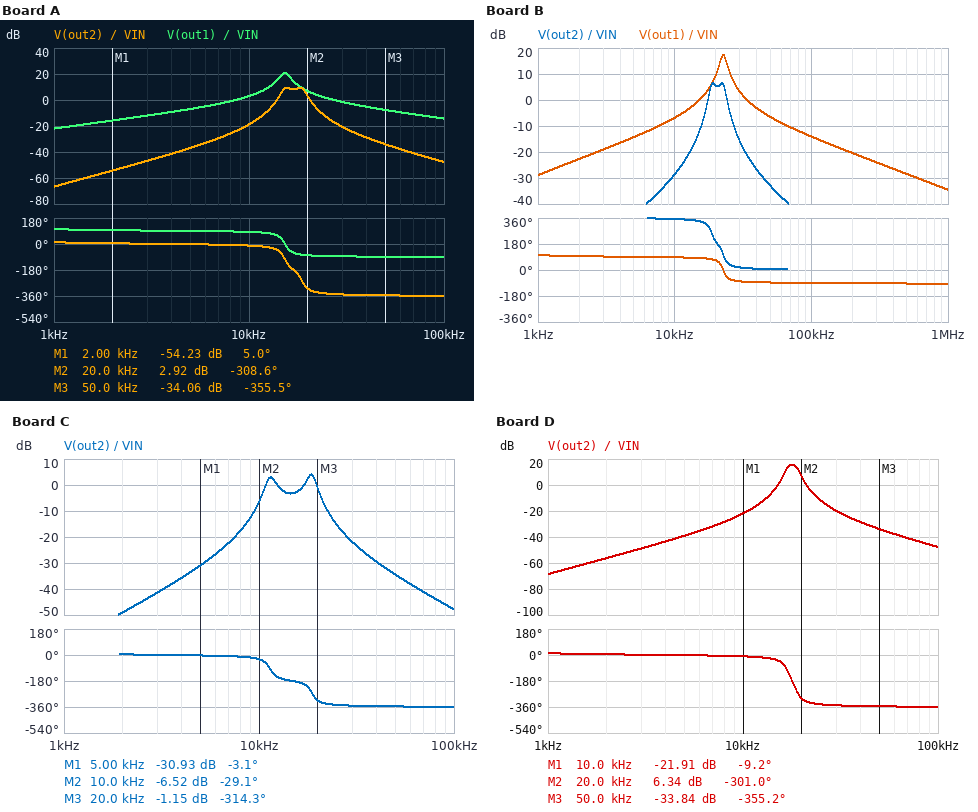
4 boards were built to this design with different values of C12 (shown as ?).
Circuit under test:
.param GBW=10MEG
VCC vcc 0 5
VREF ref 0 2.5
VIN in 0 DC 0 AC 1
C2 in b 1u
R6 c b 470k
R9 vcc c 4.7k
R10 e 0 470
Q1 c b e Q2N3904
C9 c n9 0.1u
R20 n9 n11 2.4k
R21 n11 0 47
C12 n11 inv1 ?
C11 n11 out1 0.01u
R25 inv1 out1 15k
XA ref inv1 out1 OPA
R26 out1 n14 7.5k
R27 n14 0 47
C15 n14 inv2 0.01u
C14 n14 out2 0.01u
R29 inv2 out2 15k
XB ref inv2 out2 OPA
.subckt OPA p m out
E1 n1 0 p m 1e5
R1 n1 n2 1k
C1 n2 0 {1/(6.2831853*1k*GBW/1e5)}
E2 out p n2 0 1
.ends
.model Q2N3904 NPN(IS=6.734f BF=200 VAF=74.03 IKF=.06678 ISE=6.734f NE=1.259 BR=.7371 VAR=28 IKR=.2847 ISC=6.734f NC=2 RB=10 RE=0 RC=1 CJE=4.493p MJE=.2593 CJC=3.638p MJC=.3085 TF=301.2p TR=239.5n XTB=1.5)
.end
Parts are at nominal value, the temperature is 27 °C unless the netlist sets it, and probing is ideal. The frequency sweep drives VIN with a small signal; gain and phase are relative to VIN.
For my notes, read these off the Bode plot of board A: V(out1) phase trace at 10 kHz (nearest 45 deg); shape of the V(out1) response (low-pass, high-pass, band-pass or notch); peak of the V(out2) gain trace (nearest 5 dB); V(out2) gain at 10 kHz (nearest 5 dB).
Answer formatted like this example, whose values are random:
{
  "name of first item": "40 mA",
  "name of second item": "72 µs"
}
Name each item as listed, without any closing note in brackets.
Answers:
{
  "V(out1) phase trace at 10 kHz": "90 deg",
  "shape of the V(out1) response": "band-pass",
  "peak of the V(out2) gain trace": "10 dB",
  "V(out2) gain at 10 kHz": "-20 dB"
}
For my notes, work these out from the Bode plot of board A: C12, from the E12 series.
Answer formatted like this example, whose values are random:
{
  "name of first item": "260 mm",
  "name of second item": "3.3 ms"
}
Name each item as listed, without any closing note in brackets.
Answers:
{
  "C12, from the E12 series": "15 nF"
}
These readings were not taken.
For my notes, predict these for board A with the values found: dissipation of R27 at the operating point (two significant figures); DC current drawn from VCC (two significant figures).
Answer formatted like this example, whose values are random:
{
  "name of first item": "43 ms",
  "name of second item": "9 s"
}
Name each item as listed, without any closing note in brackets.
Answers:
{
  "dissipation of R27 at the operating point": "5.2 µW",
  "DC current drawn from VCC": "420 µA"
}
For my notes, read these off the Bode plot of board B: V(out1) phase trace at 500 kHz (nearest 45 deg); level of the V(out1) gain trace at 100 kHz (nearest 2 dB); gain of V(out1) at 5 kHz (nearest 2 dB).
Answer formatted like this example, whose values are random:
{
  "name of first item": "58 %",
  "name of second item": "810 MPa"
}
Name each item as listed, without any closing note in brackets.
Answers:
{
  "V(out1) phase trace at 500 kHz": "-90 deg",
  "level of the V(out1) gain trace at 100 kHz": "-14 dB",
  "gain of V(out1) at 5 kHz": "-14 dB"
}
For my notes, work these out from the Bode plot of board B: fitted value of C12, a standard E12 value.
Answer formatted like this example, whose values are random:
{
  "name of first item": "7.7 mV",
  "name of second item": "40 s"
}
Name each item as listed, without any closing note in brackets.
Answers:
{
  "fitted value of C12, a standard E12 value": "6.8 nF"
}
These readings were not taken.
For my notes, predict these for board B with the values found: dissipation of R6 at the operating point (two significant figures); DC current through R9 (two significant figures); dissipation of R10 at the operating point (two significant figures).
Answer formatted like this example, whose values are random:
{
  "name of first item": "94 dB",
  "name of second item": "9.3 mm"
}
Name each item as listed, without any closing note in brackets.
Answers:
{
  "dissipation of R6 at the operating point": "10 µW",
  "DC current through R9": "420 µA",
  "dissipation of R10 at the operating point": "84 µW"
}
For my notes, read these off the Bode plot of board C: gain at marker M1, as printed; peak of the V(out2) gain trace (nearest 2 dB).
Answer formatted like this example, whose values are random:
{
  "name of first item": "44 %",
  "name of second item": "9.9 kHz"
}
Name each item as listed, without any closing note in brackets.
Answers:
{
  "gain at marker M1, as printed": "-30.93 dB",
  "peak of the V(out2) gain trace": "4 dB"
}
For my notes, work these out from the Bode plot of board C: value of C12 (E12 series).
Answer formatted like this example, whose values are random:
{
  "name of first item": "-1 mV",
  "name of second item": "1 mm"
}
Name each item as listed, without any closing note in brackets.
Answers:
{
  "value of C12": "27 nF"
}
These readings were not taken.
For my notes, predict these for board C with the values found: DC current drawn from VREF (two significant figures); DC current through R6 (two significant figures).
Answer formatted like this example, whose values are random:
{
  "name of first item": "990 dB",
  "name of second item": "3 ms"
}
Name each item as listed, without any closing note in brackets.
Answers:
{
  "DC current drawn from VREF": "330 µA",
  "DC current through R6": "4.6 µA"
}
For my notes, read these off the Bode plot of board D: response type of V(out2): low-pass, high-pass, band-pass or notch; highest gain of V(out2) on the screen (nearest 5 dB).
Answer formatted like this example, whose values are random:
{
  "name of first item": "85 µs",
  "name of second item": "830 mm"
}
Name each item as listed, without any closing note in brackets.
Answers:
{
  "response type of V(out2): low-pass, high-pass, band-pass or notch": "band-pass",
  "highest gain of V(out2) on the screen": "15 dB"
}
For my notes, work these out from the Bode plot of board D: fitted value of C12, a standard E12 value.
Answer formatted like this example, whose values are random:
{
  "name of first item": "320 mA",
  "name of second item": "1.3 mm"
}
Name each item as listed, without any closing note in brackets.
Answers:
{
  "fitted value of C12, a standard E12 value": "12 nF"
}
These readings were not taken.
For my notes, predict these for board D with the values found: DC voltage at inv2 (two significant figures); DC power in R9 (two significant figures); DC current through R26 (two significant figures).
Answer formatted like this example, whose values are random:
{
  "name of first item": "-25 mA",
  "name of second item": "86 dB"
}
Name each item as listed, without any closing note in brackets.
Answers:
{
  "DC voltage at inv2": "2.5 V",
  "DC power in R9": "840 µW",
  "DC current through R26": "330 µA"
}
